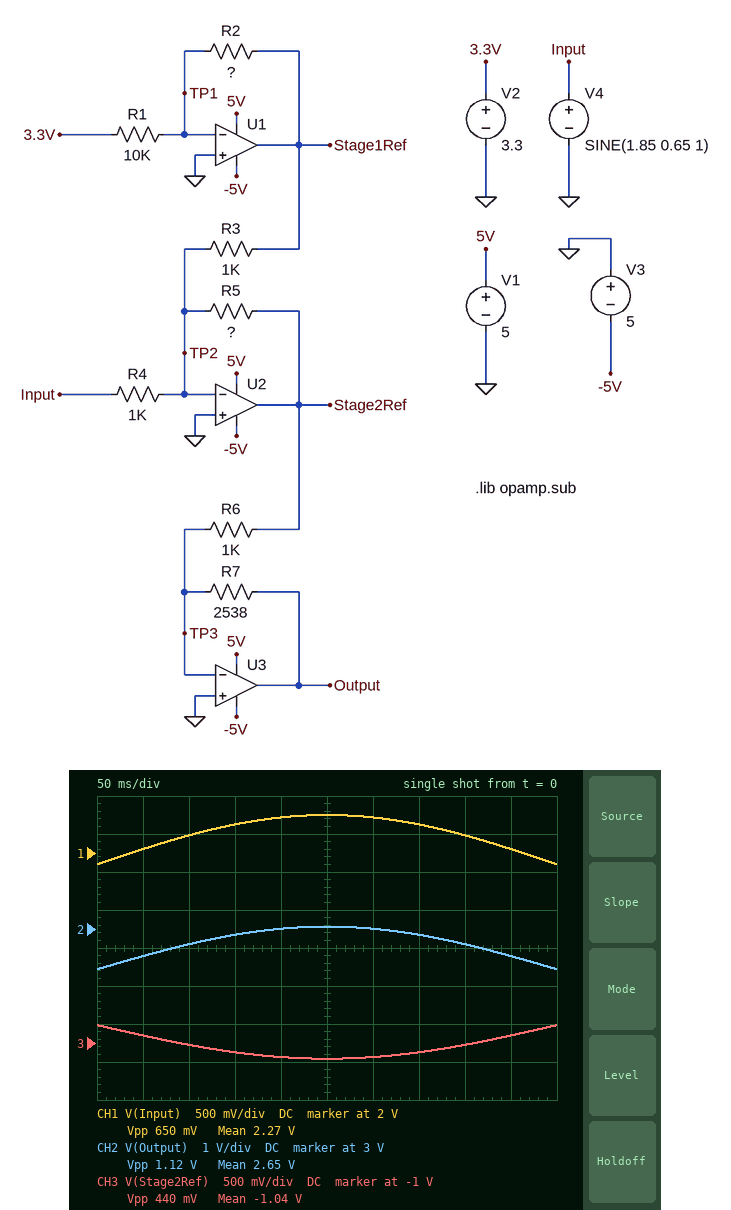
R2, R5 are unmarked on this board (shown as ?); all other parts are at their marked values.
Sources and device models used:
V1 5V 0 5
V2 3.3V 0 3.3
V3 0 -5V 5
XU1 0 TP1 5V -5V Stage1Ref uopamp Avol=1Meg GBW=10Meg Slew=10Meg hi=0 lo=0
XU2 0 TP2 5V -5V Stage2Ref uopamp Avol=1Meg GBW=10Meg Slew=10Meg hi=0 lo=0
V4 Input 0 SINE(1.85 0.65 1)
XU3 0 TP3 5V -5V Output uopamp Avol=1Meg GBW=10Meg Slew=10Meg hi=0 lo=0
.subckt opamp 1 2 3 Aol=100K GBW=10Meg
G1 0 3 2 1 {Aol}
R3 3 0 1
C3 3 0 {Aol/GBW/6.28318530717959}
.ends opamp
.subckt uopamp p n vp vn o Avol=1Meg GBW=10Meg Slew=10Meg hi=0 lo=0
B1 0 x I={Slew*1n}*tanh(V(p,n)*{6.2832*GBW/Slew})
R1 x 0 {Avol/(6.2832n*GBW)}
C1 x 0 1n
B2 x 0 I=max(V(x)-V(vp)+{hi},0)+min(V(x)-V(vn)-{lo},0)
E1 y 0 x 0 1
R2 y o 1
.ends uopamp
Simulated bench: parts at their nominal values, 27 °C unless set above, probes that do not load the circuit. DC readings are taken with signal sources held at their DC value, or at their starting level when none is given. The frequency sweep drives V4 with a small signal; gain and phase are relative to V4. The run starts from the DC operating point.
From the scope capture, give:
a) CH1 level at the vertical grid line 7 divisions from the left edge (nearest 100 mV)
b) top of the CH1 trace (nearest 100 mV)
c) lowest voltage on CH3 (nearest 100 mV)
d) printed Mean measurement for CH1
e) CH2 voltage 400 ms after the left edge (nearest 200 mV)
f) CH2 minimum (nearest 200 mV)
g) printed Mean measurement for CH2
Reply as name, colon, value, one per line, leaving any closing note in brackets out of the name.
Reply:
CH1 level at the vertical grid line 7 divisions from the left edge: 2.4 V
top of the CH1 trace: 2.5 V
lowest voltage on CH3: -1.2 V
printed Mean measurement for CH1: 2.27 V
CH2 voltage 400 ms after the left edge: 2.6 V
CH2 minimum: 2.0 V
printed Mean measurement for CH2: 2.65 V
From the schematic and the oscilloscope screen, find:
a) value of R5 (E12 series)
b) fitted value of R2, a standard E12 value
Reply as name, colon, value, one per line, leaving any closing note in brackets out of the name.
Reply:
value of R5: 680 Ω
fitted value of R2, a standard E12 value: 2.2 kΩ
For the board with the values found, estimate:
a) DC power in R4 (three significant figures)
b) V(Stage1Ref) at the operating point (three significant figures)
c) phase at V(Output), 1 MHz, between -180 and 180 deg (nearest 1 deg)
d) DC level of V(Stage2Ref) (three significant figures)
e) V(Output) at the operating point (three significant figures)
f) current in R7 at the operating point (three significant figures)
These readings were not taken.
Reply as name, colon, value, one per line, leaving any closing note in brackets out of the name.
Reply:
DC power in R4: 3.42 mW
V(Stage1Ref) at the operating point: -726 mV
phase at V(Output), 1 MHz, between -180 and 180 deg: -33 deg
DC level of V(Stage2Ref): -764 mV
V(Output) at the operating point: 1.94 V
current in R7 at the operating point: 764 µA
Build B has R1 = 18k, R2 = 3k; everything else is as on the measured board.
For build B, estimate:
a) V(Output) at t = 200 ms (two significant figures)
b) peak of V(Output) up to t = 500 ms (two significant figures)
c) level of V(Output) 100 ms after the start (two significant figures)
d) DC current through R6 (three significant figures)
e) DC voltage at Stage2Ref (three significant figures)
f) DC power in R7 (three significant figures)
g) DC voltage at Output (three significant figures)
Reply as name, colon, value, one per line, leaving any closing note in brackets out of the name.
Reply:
V(Output) at t = 200 ms: 3.3 V
peak of V(Output) up to t = 500 ms: 3.4 V
level of V(Output) 100 ms after the start: 2.9 V
DC current through R6: 884 µA
DC voltage at Stage2Ref: -884 mV
DC power in R7: 1.98 mW
DC voltage at Output: 2.24 V
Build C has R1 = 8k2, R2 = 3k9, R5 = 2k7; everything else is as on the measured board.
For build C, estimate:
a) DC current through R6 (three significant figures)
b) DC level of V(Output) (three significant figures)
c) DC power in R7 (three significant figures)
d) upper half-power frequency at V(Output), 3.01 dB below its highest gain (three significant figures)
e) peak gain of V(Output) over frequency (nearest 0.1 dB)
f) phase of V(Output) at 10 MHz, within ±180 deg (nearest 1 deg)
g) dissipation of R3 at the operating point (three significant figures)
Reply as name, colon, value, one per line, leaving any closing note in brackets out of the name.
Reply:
DC current through R6: 757 µA
DC level of V(Output): 1.92 V
DC power in R7: 1.46 mW
upper half-power frequency at V(Output), 3.01 dB below its highest gain: 1.27 MHz
peak gain of V(Output) over frequency: 16.7 dB
phase of V(Output) at 10 MHz, within ±180 deg: -155 deg
dissipation of R3 at the operating point: 2.46 mW
